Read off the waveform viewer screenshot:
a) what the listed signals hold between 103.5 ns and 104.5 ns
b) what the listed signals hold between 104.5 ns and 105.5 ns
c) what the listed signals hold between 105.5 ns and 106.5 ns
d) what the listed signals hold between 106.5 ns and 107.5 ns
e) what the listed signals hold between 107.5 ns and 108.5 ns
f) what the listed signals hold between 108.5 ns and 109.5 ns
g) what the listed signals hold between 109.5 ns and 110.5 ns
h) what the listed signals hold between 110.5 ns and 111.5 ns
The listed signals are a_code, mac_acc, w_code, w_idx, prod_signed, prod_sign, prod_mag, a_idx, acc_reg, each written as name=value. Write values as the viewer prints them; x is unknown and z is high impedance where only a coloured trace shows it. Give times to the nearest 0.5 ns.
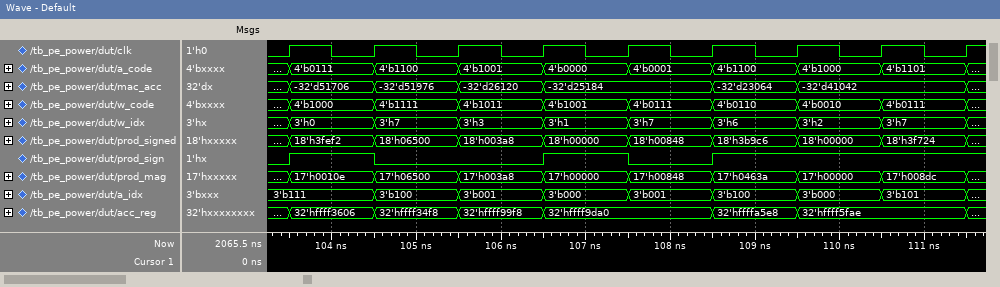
a_code=4'b0111, mac_acc=-32'd51706, w_code=4'b1000, w_idx=3'h0, prod_signed=18'h3fef2, prod_sign=1, prod_mag=17'h0010e, a_idx=3'b111, acc_reg=32'hffff3606
a_code=4'b1100, mac_acc=-32'd51976, w_code=4'b1111, w_idx=3'h7, prod_signed=18'h06500, prod_sign=0, prod_mag=17'h06500, a_idx=3'b100, acc_reg=32'hffff34f8
a_code=4'b1001, mac_acc=-32'd26120, w_code=4'b1011, w_idx=3'h3, prod_signed=18'h003a8, prod_sign=0, prod_mag=17'h003a8, a_idx=3'b001, acc_reg=32'hffff99f8
a_code=4'b0000, mac_acc=-32'd25184, w_code=4'b1001, w_idx=3'h1, prod_signed=18'h00000, prod_sign=1, prod_mag=17'h00000, a_idx=3'b000, acc_reg=32'hffff9da0
a_code=4'b0001, mac_acc=-32'd25184, w_code=4'b0111, w_idx=3'h7, prod_signed=18'h00848, prod_sign=0, prod_mag=17'h00848, a_idx=3'b001, acc_reg=32'hffff9da0
a_code=4'b1100, mac_acc=-32'd23064, w_code=4'b0110, w_idx=3'h6, prod_signed=18'h3b9c6, prod_sign=1, prod_mag=17'h0463a, a_idx=3'b100, acc_reg=32'hffffa5e8
a_code=4'b1000, mac_acc=-32'd41042, w_code=4'b0010, w_idx=3'h2, prod_signed=18'h00000, prod_sign=1, prod_mag=17'h00000, a_idx=3'b000, acc_reg=32'hffff5fae
a_code=4'b1101, mac_acc=-32'd41042, w_code=4'b0111, w_idx=3'h7, prod_signed=18'h3f724, prod_sign=1, prod_mag=17'h008dc, a_idx=3'b101, acc_reg=32'hffff5fae
